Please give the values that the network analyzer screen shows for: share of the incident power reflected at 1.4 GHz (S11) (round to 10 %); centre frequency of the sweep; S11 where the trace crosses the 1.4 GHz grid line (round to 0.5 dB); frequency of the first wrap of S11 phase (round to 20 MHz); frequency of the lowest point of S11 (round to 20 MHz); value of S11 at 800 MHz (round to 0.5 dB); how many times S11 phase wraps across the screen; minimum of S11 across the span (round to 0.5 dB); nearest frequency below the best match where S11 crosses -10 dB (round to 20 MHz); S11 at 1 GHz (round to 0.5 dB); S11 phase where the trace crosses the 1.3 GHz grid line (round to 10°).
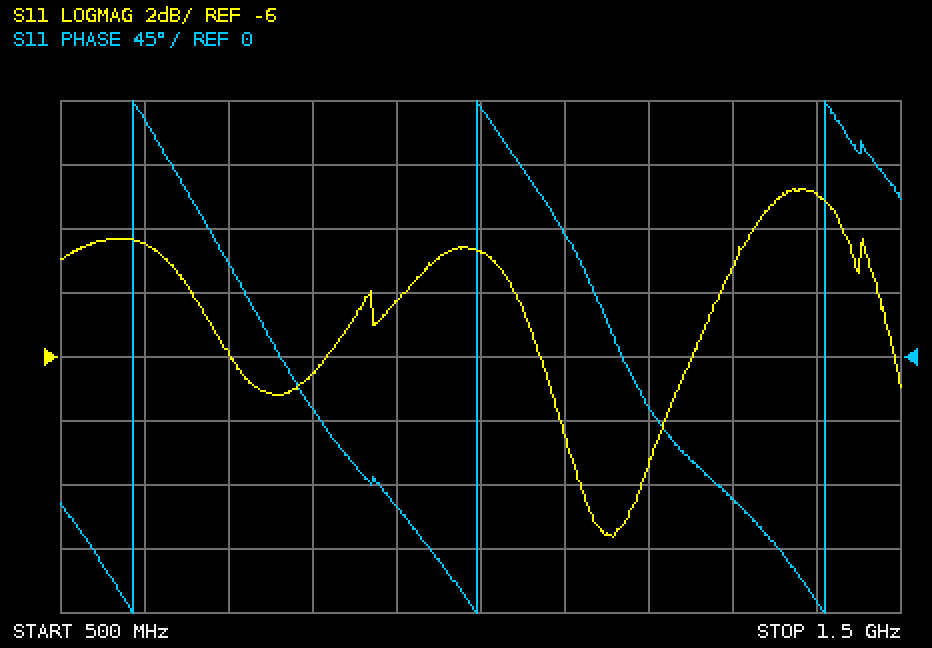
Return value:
80 %
1 GHz
-1.0 dB
580 MHz
1.16 GHz
-6.5 dB
3
-11.5 dB
1.12 GHz
-2.5 dB
-100°
